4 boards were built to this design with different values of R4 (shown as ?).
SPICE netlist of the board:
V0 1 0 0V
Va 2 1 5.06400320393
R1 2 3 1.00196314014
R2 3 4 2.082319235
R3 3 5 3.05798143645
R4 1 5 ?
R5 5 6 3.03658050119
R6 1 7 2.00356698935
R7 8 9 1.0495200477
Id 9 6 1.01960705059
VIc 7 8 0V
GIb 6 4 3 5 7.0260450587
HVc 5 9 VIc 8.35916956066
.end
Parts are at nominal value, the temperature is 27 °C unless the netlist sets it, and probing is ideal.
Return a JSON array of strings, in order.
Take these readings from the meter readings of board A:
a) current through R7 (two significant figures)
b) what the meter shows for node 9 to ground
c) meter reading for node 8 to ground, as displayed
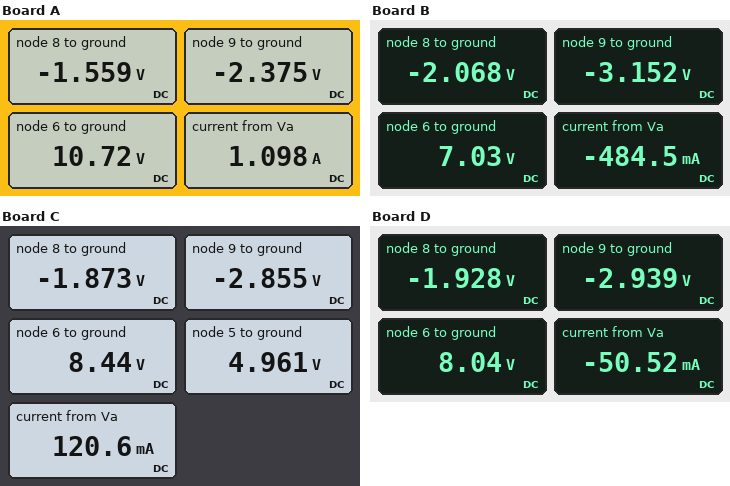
["780 mA", "-2.375 V", "-1.559 V"]
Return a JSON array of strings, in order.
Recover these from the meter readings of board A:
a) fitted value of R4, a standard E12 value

["2.2 Ω"]
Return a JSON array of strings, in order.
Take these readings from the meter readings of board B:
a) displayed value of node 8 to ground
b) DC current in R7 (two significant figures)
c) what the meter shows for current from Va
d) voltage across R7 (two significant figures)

["-2.068 V", "1.0 A", "-484.5 mA", "1.1 V"]
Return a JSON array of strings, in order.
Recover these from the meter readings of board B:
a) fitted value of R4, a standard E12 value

["10 Ω"]
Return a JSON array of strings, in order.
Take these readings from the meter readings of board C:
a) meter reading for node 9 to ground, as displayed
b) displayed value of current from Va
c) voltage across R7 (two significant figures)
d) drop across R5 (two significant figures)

["-2.855 V", "120.6 mA", "980 mV", "3.5 V"]
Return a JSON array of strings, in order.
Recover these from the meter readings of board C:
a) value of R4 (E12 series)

["4.7 Ω"]
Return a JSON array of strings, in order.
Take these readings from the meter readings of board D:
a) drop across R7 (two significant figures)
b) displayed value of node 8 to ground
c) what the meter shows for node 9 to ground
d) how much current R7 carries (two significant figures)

["1.0 V", "-1.928 V", "-2.939 V", "960 mA"]
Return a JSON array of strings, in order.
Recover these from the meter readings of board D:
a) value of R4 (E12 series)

["5.6 Ω"]
